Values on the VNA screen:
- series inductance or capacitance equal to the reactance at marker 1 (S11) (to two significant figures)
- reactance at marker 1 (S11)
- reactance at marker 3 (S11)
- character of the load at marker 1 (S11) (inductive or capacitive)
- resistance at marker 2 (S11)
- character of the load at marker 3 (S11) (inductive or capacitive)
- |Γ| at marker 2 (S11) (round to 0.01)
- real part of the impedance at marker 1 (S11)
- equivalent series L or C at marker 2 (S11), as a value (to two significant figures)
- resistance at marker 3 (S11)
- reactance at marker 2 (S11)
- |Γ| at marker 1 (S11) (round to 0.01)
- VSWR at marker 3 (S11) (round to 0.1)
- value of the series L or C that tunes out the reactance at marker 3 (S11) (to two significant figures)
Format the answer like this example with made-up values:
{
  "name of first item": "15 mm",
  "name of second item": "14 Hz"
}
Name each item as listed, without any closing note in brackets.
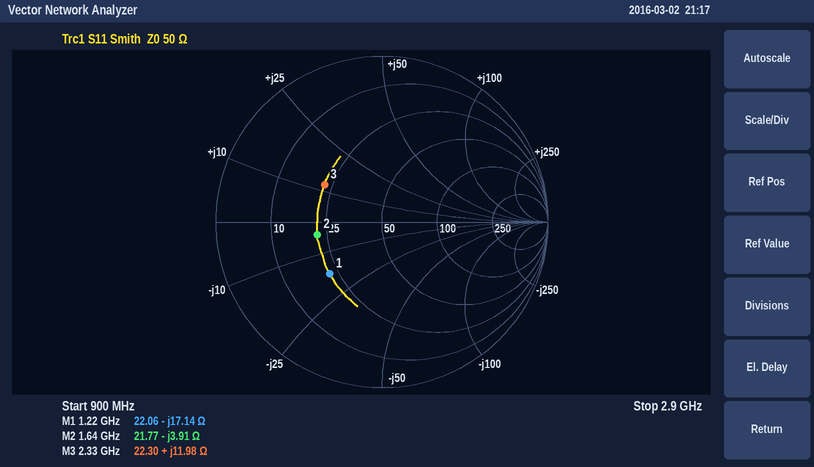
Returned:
{
  "series inductance or capacitance equal to the reactance at marker 1 (S11)": "7.6 pF",
  "reactance at marker 1": "-17.14 Ω",
  "reactance at marker 3": "+11.98 Ω",
  "character of the load at marker 1 (S11)": "capacitive",
  "resistance at marker 2": "21.77 Ω",
  "character of the load at marker 3 (S11)": "inductive",
  "|Γ| at marker 2 (S11)": "0.40",
  "real part of the impedance at marker 1": "22.06 Ω",
  "equivalent series L or C at marker 2 (S11), as a value": "25 pF",
  "resistance at marker 3": "22.30 Ω",
  "reactance at marker 2": "-3.91 Ω",
  "|Γ| at marker 1 (S11)": "0.44",
  "VSWR at marker 3 (S11)": "2.4",
  "value of the series L or C that tunes out the reactance at marker 3 (S11)": "5.7 pF"
}
